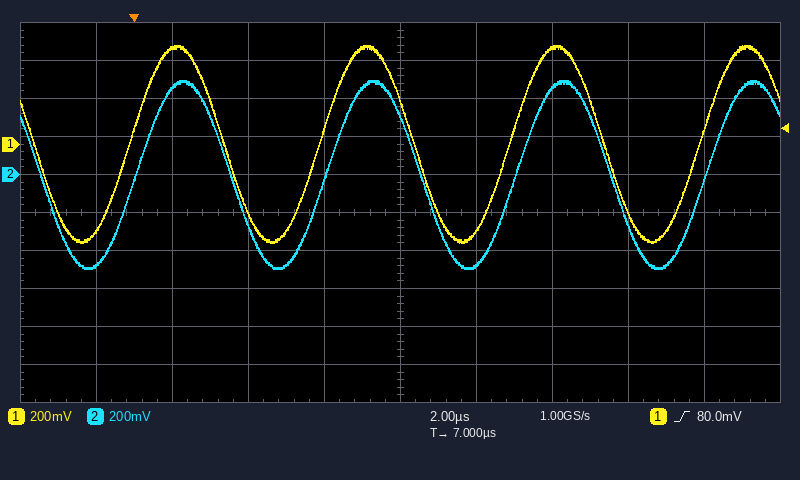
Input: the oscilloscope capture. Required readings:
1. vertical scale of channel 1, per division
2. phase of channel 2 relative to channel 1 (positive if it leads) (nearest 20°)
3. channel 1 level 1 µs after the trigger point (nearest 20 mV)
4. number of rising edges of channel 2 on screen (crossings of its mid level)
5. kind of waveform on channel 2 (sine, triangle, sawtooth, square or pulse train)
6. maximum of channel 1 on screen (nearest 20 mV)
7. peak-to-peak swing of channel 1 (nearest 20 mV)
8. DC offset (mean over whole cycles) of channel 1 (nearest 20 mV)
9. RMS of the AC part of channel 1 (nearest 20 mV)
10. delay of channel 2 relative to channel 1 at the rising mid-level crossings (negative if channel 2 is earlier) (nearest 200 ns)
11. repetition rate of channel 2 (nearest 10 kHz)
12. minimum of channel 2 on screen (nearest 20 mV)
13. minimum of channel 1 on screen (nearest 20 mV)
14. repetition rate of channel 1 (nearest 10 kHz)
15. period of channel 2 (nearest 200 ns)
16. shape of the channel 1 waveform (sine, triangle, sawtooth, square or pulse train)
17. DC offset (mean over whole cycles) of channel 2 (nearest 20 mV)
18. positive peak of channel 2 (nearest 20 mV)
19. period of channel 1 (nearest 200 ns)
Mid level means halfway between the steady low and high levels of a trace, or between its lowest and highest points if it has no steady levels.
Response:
200 mV
-20°
500 mV
4
sine
520 mV
1.04 V
0 mV
360 mV
+200 ns
200 kHz
-500 mV
-520 mV
200 kHz
5.0 µs
sine
0 mV
500 mV
5.0 µs
